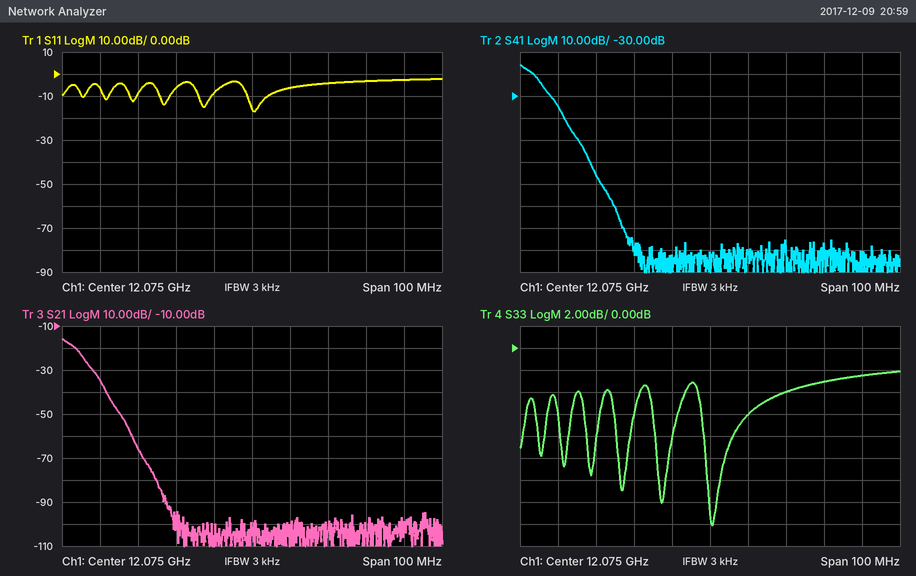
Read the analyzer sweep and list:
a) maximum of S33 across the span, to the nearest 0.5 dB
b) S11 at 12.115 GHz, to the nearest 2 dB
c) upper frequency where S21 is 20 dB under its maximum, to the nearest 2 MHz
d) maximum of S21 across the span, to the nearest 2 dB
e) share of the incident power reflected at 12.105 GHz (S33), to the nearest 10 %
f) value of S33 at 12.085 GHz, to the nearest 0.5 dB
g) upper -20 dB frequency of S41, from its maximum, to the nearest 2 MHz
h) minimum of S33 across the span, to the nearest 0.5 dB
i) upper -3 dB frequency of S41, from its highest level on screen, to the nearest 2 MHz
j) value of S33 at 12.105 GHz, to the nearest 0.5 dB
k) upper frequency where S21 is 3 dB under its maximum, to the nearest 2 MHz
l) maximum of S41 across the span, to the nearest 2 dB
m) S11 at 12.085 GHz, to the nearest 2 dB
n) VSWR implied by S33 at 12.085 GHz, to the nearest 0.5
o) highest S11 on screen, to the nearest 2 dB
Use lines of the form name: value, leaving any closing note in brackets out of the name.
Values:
maximum of S33 across the span, to the nearest 0.5 dB: -2.0 dB
S11 at 12.115 GHz, to the nearest 2 dB: -2 dB
upper frequency where S21 is 20 dB under its maximum, to the nearest 2 MHz: 12.036 GHz
maximum of S21 across the span, to the nearest 2 dB: -16 dB
share of the incident power reflected at 12.105 GHz (S33), to the nearest 10 %: 50 %
value of S33 at 12.085 GHz, to the nearest 0.5 dB: -6.0 dB
upper -20 dB frequency of S41, from its maximum, to the nearest 2 MHz: 12.036 GHz
minimum of S33 across the span, to the nearest 0.5 dB: -16.0 dB
upper -3 dB frequency of S41, from its highest level on screen, to the nearest 2 MHz: 12.028 GHz
value of S33 at 12.105 GHz, to the nearest 0.5 dB: -3.0 dB
upper frequency where S21 is 3 dB under its maximum, to the nearest 2 MHz: 12.028 GHz
maximum of S41 across the span, to the nearest 2 dB: -16 dB
S11 at 12.085 GHz, to the nearest 2 dB: -6 dB
VSWR implied by S33 at 12.085 GHz, to the nearest 0.5: 3.0
highest S11 on screen, to the nearest 2 dB: -2 dB
